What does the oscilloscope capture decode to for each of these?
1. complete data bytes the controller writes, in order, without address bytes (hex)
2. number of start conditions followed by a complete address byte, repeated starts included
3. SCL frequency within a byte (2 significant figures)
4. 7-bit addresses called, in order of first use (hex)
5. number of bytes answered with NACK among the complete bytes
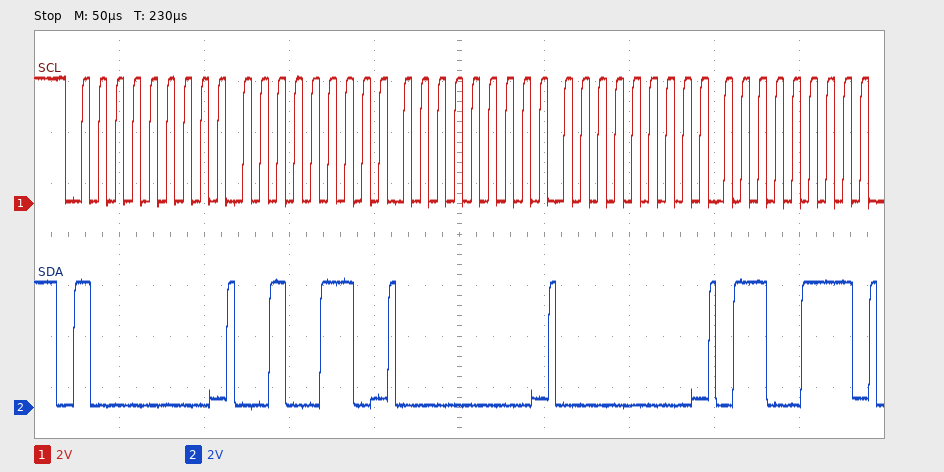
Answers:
26 00 00 67
1
100 kHz
0x40
0
